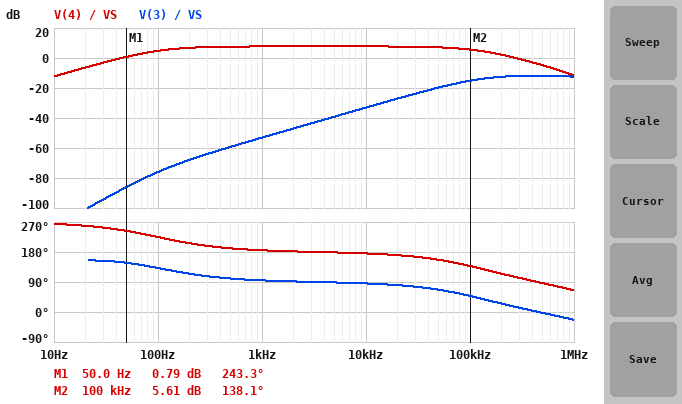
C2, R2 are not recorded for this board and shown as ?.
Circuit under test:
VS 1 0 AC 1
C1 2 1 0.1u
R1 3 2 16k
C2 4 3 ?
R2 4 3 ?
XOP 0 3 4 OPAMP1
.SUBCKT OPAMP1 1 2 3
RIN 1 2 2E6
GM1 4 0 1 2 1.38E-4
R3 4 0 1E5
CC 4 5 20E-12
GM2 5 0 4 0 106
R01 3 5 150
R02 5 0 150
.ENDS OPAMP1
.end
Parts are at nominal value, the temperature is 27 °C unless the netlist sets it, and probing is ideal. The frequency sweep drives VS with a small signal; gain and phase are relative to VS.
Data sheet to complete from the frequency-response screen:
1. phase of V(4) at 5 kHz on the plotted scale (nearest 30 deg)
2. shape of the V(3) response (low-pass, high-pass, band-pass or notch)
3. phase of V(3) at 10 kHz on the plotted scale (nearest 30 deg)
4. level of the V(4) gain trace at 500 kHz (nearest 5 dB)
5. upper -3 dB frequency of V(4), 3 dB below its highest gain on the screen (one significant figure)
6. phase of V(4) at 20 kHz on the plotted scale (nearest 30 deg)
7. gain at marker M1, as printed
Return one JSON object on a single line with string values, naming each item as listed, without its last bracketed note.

{"phase of V(4) at 5 kHz on the plotted scale": "180 deg", "shape of the V(3) response": "high-pass", "phase of V(3) at 10 kHz on the plotted scale": "90 deg", "level of the V(4) gain trace at 500 kHz": "-5 dB", "upper -3 dB frequency of V(4), 3 dB below its highest gain on the screen": "100 kHz", "phase of V(4) at 20 kHz on the plotted scale": "180 deg", "gain at marker M1, as printed": "0.79 dB"}
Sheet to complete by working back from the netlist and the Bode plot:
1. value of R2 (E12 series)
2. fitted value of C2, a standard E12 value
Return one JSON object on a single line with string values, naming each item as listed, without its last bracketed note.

{"value of R2": "39 kΩ", "fitted value of C2, a standard E12 value": "22 pF"}
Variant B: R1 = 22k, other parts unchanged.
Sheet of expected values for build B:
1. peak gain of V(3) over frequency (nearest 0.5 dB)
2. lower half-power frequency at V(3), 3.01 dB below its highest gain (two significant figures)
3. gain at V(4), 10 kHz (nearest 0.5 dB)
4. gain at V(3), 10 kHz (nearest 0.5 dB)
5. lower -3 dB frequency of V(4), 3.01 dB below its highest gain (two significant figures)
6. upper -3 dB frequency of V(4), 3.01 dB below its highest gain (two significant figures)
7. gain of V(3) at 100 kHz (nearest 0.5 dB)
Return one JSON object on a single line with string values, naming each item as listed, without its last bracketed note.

{"peak gain of V(3) over frequency": "-14.0 dB", "lower half-power frequency at V(3), 3.01 dB below its highest gain": "120 kHz", "gain at V(4), 10 kHz": "5.0 dB", "gain at V(3), 10 kHz": "-36.0 dB", "lower -3 dB frequency of V(4), 3.01 dB below its highest gain": "72 Hz", "upper -3 dB frequency of V(4), 3.01 dB below its highest gain": "140 kHz", "gain of V(3) at 100 kHz": "-17.5 dB"}
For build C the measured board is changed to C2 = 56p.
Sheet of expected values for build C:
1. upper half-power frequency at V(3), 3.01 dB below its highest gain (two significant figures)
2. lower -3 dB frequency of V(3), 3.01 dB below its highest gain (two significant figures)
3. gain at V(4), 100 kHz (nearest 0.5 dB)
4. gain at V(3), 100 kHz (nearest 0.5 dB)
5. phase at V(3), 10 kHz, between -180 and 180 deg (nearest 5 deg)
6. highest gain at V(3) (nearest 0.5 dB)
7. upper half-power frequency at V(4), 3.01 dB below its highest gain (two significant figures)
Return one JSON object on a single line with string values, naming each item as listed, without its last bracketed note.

{"upper half-power frequency at V(3), 3.01 dB below its highest gain": "1.4 MHz", "lower -3 dB frequency of V(3), 3.01 dB below its highest gain": "57 kHz", "gain at V(4), 100 kHz": "2.0 dB", "gain at V(3), 100 kHz": "-18.5 dB", "phase at V(3), 10 kHz, between -180 and 180 deg": "80 deg", "highest gain at V(3)": "-17.5 dB", "upper half-power frequency at V(4), 3.01 dB below its highest gain": "62 kHz"}
